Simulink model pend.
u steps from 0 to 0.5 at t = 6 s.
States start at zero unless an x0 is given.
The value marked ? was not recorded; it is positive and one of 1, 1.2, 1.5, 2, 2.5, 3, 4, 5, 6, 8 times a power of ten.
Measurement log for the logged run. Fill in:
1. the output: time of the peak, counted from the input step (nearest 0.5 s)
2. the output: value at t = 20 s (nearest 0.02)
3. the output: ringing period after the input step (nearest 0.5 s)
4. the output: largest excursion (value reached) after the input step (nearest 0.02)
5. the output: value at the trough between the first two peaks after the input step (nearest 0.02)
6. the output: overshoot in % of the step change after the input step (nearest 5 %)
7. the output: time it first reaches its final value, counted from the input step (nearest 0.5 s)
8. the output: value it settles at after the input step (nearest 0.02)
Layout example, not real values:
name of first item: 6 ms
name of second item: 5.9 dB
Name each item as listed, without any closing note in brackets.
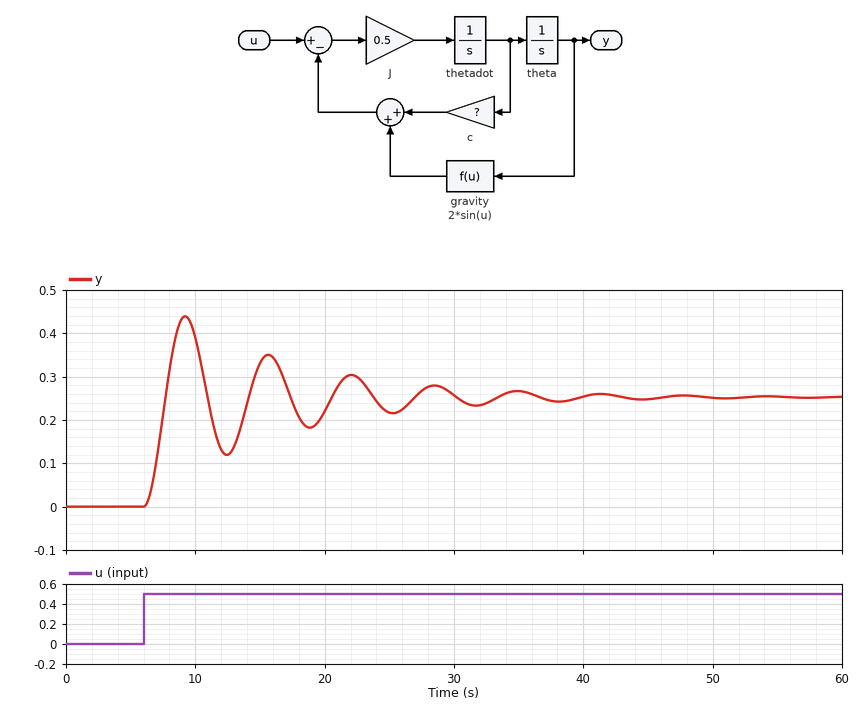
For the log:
the output: time of the peak, counted from the input step: 3.0 s
the output: value at t = 20 s: 0.22
the output: ringing period after the input step: 6.5 s
the output: largest excursion (value reached) after the input step: 0.44
the output: value at the trough between the first two peaks after the input step: 0.12
the output: overshoot in % of the step change after the input step: 75 %
the output: time it first reaches its final value, counted from the input step: 1.5 s
the output: value it settles at after the input step: 0.26
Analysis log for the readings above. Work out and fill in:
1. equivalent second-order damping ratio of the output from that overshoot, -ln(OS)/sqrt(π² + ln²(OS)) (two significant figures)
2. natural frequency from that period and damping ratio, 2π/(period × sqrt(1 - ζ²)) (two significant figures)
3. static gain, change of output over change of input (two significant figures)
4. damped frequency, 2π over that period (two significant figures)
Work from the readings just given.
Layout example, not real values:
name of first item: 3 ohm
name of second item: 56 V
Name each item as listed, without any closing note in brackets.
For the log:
equivalent second-order damping ratio of the output from that overshoot, -ln(OS)/sqrt(π² + ln²(OS)): 0.091
natural frequency from that period and damping ratio, 2π/(period × sqrt(1 - ζ²)): 0.97 rad/s
static gain, change of output over change of input: 0.52
damped frequency, 2π over that period: 0.97 rad/s
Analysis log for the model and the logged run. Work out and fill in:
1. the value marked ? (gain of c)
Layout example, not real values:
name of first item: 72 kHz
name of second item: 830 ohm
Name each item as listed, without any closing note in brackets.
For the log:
the value marked ?: 0.4
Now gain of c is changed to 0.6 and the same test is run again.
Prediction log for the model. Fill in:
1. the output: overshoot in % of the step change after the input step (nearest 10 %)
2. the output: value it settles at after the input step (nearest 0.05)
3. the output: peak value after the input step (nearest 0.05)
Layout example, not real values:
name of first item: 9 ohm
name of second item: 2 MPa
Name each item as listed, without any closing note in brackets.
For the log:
the output: overshoot in % of the step change after the input step: 60 %
the output: value it settles at after the input step: 0.25
the output: peak value after the input step: 0.40
